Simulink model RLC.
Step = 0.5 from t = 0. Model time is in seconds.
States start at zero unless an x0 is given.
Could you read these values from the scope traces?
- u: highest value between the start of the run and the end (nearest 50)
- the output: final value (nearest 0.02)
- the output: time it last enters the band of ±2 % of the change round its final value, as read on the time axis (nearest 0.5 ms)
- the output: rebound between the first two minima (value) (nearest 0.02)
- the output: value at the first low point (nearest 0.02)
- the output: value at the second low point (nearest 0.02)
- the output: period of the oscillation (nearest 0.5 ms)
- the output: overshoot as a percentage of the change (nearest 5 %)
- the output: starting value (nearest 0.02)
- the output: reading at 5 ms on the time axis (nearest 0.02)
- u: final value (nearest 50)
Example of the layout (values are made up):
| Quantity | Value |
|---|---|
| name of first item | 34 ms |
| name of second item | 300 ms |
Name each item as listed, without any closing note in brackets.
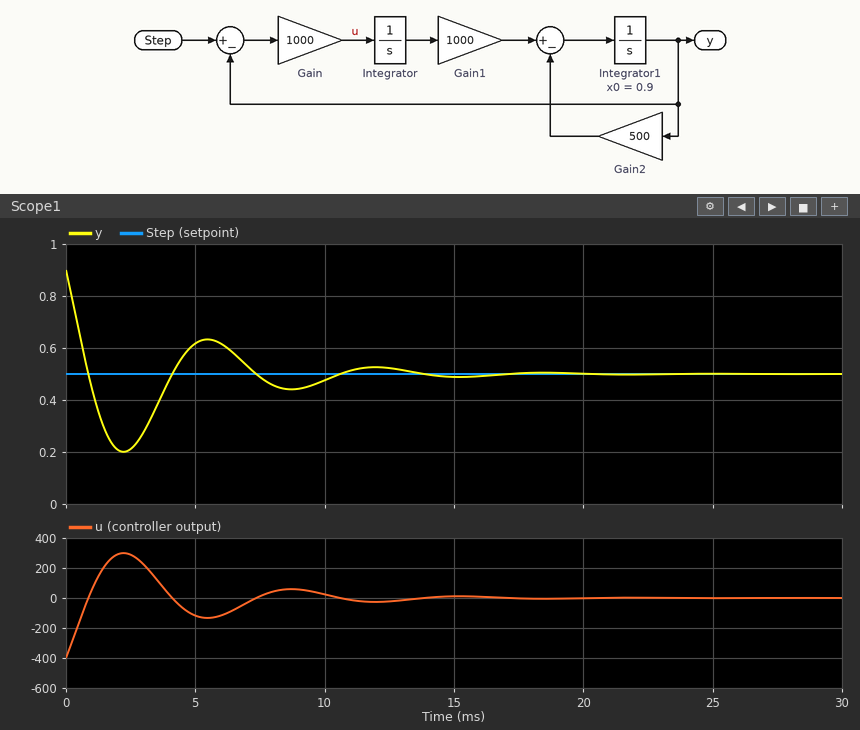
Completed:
| Quantity | Value |
|---|---|
| u: highest value between the start of the run and the end | 300 |
| the output: final value | 0.50 |
| the output: time it last enters the band of ±2 % of the change round its final value, as read on the time axis | 16.0 ms |
| the output: rebound between the first two minima (value) | 0.64 |
| the output: value at the first low point | 0.20 |
| the output: value at the second low point | 0.44 |
| the output: period of the oscillation | 6.5 ms |
| the output: overshoot as a percentage of the change | 75 % |
| the output: starting value | 0.90 |
| the output: reading at 5 ms on the time axis | 0.62 |
| u: final value | 0 |
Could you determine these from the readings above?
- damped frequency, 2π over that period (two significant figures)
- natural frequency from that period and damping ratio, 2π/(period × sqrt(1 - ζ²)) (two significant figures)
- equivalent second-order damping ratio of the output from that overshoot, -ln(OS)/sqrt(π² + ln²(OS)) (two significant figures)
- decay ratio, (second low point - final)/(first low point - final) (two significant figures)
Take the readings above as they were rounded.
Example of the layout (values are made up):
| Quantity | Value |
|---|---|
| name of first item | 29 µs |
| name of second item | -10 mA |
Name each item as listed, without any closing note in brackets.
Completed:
| Quantity | Value |
|---|---|
| damped frequency, 2π over that period | 0.97 rad/ms |
| natural frequency from that period and damping ratio, 2π/(period × sqrt(1 - ζ²)) | 0.97 rad/ms |
| equivalent second-order damping ratio of the output from that overshoot, -ln(OS)/sqrt(π² + ln²(OS)) | 0.091 |
| decay ratio, (second low point - final)/(first low point - final) | 0.20 |
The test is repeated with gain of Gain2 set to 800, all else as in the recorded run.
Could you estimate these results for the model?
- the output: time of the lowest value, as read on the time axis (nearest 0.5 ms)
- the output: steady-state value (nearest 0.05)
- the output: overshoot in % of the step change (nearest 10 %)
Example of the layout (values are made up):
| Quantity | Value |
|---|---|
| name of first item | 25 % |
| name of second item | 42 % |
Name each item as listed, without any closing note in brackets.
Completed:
| Quantity | Value |
|---|---|
| the output: time of the lowest value, as read on the time axis | 2.0 ms |
| the output: steady-state value | 0.50 |
| the output: overshoot in % of the step change | 80 % |
